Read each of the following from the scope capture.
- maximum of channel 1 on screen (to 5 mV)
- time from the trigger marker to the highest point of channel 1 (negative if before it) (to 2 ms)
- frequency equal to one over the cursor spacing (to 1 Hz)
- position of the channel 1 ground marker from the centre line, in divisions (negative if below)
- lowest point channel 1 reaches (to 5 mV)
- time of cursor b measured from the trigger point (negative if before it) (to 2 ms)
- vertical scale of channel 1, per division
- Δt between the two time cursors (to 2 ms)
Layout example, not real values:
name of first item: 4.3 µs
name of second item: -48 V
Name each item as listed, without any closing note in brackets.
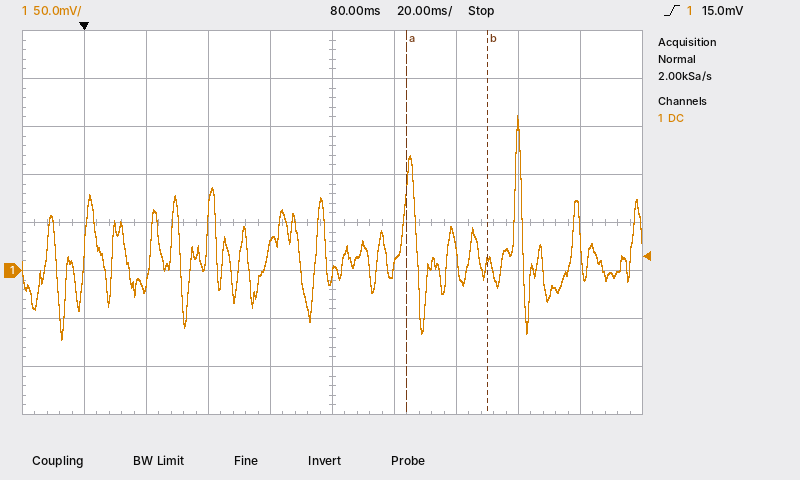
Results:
maximum of channel 1 on screen: 160 mV
time from the trigger marker to the highest point of channel 1 (negative if before it): +140 ms
frequency equal to one over the cursor spacing: 38 Hz
position of the channel 1 ground marker from the centre line, in divisions: -1.0 div
lowest point channel 1 reaches: -70 mV
time of cursor b measured from the trigger point (negative if before it): +130 ms
vertical scale of channel 1, per division: 50 mV
Δt between the two time cursors: 26 ms
